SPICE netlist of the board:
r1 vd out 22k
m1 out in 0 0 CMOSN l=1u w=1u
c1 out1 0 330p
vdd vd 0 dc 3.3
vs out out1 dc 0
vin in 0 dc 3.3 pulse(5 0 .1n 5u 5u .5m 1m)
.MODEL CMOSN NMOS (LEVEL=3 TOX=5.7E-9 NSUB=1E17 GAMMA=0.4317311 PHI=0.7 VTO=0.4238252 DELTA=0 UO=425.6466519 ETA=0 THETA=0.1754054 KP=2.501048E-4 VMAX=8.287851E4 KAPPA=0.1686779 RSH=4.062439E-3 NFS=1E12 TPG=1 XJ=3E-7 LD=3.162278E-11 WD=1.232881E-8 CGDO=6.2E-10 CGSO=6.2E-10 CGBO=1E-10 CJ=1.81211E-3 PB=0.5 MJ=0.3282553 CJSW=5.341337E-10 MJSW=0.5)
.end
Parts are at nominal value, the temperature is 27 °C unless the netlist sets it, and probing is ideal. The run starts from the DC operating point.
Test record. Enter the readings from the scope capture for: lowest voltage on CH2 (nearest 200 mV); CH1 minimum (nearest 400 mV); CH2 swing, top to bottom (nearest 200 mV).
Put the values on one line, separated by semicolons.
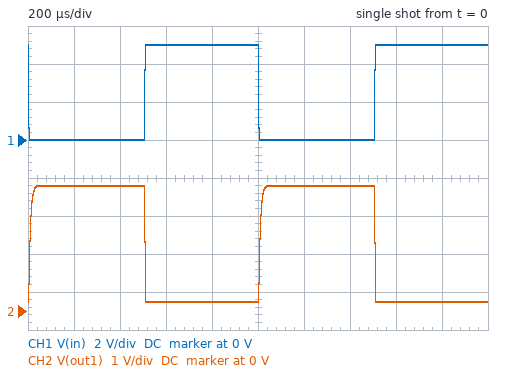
200 mV; 0 V; 3.0 V
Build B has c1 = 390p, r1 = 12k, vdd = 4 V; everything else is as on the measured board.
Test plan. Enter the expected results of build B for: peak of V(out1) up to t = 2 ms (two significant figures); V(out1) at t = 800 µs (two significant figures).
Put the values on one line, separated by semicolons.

4.0 V; 570 mV
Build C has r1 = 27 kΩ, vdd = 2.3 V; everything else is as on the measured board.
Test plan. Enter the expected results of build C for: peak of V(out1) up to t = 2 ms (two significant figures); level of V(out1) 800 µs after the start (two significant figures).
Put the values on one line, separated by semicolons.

2.3 V; 140 mV
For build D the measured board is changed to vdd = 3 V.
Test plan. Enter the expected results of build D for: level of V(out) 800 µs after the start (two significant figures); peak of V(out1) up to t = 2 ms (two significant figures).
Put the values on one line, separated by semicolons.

220 mV; 3.0 V
